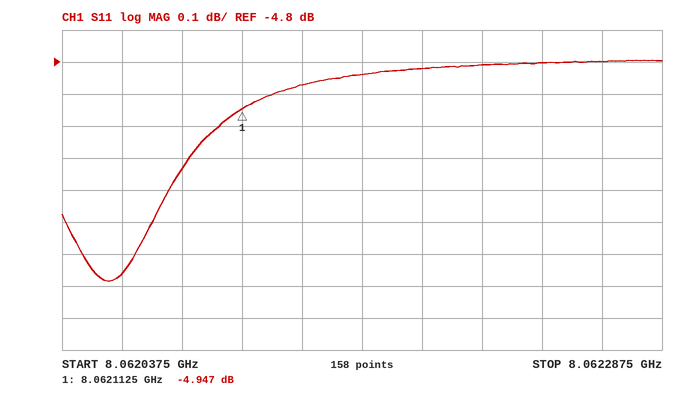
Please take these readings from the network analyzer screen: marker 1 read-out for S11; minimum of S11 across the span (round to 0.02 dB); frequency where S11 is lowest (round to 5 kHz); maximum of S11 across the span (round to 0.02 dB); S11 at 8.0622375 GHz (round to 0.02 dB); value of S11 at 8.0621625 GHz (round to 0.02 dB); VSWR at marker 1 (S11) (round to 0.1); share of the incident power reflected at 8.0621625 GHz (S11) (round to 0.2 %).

-4.947 dB
-5.48 dB
8.062055 GHz
-4.80 dB
-4.80 dB
-4.84 dB
3.6
32.8 %
